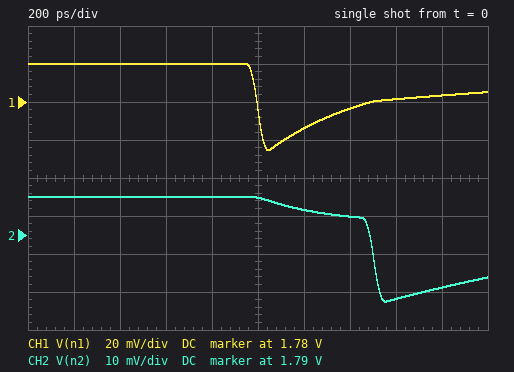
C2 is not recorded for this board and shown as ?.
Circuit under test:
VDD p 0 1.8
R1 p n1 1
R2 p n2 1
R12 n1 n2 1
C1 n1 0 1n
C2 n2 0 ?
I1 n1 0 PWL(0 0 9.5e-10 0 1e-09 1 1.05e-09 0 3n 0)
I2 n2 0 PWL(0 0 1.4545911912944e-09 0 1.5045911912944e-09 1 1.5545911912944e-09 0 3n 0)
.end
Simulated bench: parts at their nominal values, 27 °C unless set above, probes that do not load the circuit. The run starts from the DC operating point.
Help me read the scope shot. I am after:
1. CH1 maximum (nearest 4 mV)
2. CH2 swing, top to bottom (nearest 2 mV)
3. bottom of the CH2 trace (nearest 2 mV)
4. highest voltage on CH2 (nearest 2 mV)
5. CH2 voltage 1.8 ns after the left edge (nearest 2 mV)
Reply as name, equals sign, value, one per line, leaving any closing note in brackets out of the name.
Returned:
CH1 maximum = 1.800 V
CH2 swing, top to bottom = 28 mV
bottom of the CH2 trace = 1.772 V
highest voltage on CH2 = 1.800 V
CH2 voltage 1.8 ns after the left edge = 1.776 V
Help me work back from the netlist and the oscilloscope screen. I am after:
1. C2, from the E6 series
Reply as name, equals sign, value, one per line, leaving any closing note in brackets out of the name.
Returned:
C2, from the E6 series = 2.2 nF
